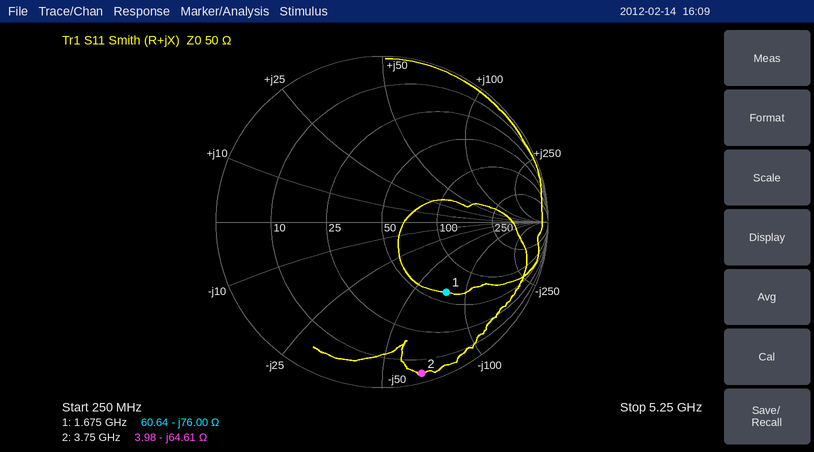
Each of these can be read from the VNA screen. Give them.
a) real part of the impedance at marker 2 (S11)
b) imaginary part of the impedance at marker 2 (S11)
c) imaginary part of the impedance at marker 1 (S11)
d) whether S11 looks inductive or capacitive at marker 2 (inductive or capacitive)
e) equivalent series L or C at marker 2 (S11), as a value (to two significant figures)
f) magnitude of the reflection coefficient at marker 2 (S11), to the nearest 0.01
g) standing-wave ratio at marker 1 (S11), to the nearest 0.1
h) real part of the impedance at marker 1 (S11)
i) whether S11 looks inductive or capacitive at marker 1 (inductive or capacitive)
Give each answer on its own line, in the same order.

3.98 Ω
-64.61 Ω
-76.00 Ω
capacitive
660 fF
0.94
3.7
60.64 Ω
capacitive
